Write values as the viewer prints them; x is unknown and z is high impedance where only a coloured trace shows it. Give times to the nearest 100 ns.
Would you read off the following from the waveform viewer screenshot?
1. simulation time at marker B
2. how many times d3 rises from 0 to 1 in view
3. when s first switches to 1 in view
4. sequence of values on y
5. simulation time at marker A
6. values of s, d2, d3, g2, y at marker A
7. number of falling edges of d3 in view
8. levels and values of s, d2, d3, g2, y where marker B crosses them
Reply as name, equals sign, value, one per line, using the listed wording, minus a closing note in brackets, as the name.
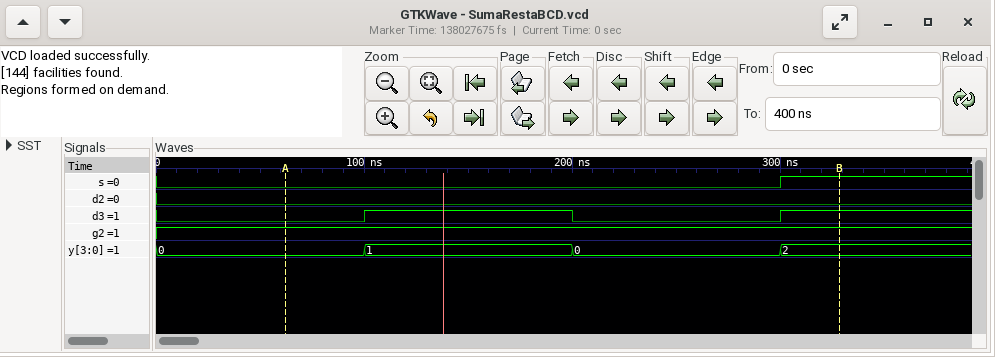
simulation time at marker B = 300 ns
how many times d3 rises from 0 to 1 in view = 2
when s first switches to 1 in view = 300 ns
sequence of values on y = 0, 1, 0, 2
simulation time at marker A = 100 ns
values of s, d2, d3, g2, y at marker A = s=0, d2=0, d3=0, g2=1, y=0
number of falling edges of d3 in view = 1
levels and values of s, d2, d3, g2, y where marker B crosses them = s=1, d2=0, d3=1, g2=1, y=2
